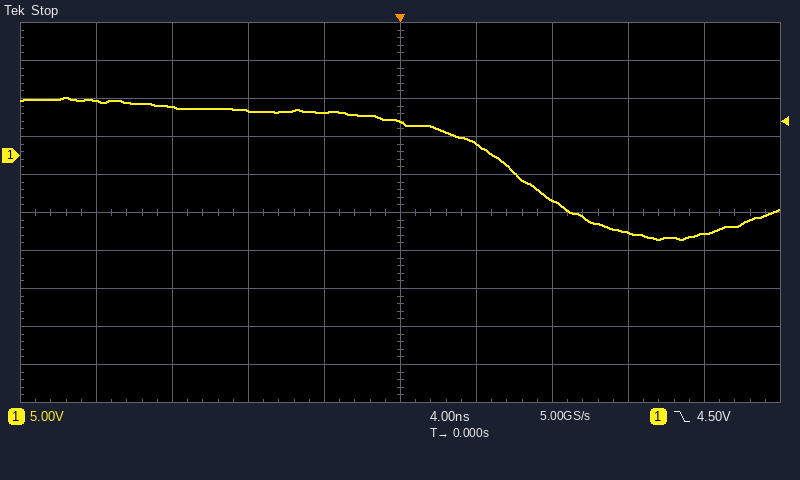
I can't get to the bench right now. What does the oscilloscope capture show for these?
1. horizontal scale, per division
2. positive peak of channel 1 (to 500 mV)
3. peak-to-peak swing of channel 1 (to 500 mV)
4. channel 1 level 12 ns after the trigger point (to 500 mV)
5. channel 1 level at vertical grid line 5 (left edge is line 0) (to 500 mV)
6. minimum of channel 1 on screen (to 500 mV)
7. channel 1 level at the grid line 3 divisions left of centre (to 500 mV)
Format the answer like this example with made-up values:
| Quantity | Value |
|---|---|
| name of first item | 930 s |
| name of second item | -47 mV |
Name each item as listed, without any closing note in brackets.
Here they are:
| Quantity | Value |
|---|---|
| horizontal scale, per division | 4 ns |
| positive peak of channel 1 | 7.5 V |
| peak-to-peak swing of channel 1 | 18.5 V |
| channel 1 level 12 ns after the trigger point | -10.0 V |
| channel 1 level at vertical grid line 5 (left edge is line 0) | 4.5 V |
| minimum of channel 1 on screen | -11.0 V |
| channel 1 level at the grid line 3 divisions left of centre | 6.5 V |
